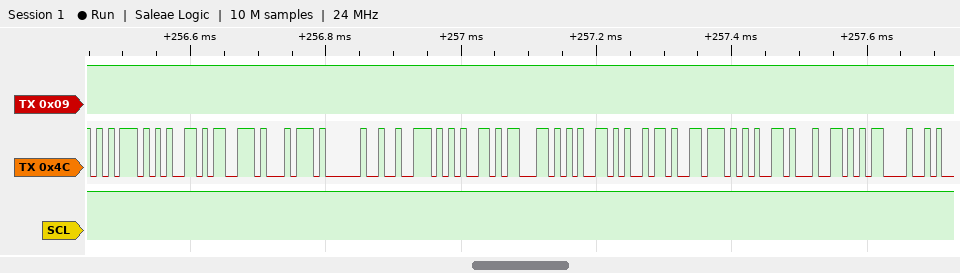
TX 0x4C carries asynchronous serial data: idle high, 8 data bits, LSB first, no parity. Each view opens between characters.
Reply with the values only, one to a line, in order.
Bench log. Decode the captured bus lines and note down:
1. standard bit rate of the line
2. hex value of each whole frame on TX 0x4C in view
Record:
115200 baud
75, 65, 73, 74, 20, 72, 65, 63, 65, 69, 76, 65, 64, 0D
